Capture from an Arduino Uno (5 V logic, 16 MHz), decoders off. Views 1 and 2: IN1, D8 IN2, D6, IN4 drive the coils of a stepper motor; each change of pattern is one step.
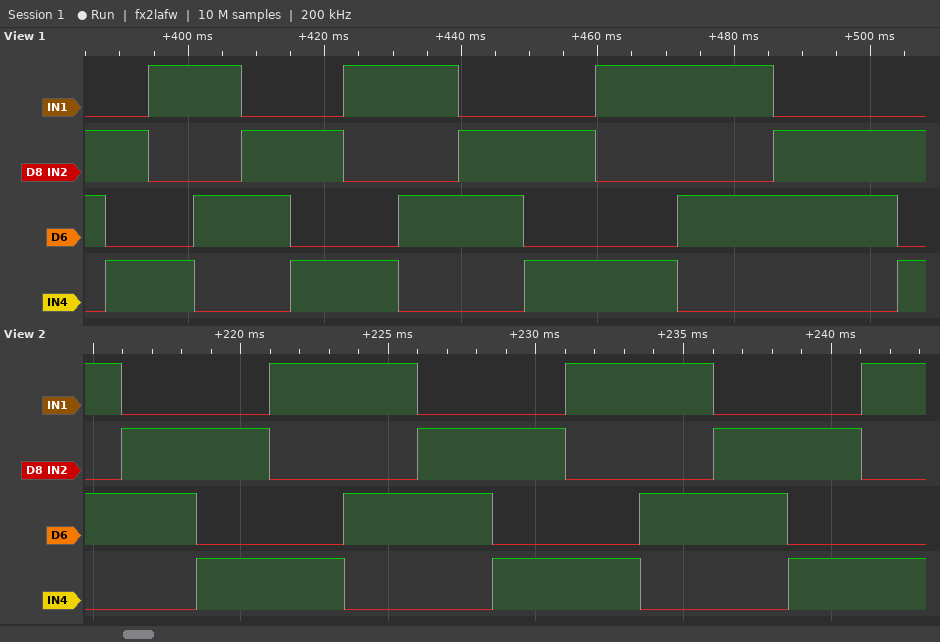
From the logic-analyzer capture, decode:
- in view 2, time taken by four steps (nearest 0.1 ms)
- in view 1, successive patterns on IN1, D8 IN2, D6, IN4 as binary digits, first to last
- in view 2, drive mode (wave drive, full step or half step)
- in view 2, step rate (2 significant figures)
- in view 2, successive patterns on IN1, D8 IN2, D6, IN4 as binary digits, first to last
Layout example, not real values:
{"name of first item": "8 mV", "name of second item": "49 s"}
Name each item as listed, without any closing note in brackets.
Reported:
{"in view 2, time taken by four steps": "10.0 ms", "in view 1, successive patterns on IN1, D8 IN2, D6, IN4 as binary digits, first to last": "0110 0101 1001 1010 0110 0101 1001 1010 0110 0101 1001 1010 0110 0101", "in view 2, drive mode": "full step", "in view 2, step rate": "400 steps/s", "in view 2, successive patterns on IN1, D8 IN2, D6, IN4 as binary digits, first to last": "1010 0110 0101 1001 1010 0110 0101 1001 1010 0110 0101 1001"}
